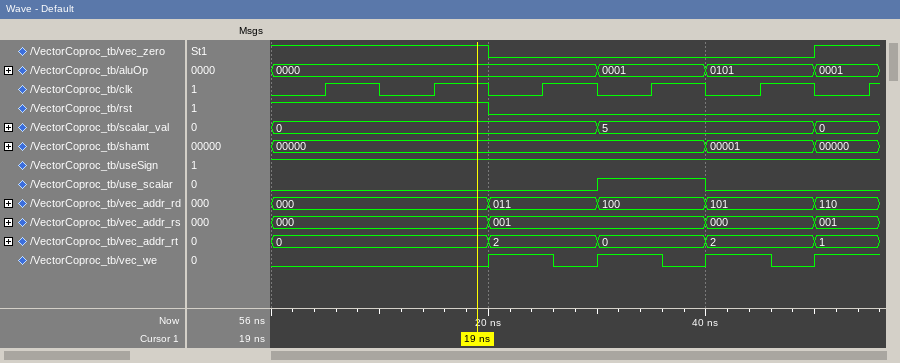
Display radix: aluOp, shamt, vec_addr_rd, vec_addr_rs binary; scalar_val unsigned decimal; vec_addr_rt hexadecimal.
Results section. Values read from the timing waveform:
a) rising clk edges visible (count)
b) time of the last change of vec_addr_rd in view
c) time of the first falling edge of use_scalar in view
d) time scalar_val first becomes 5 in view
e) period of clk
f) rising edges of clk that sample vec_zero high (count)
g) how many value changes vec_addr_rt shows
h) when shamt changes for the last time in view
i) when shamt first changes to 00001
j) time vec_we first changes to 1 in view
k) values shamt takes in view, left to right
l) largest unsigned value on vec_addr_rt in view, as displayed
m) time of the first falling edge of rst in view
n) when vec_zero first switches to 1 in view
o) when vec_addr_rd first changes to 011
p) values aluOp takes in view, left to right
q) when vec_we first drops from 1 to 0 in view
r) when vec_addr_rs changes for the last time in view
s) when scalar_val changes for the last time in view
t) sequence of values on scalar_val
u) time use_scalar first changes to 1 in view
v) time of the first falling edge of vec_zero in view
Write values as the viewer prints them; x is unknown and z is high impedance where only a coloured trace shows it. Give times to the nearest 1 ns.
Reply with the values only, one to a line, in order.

6
50 ns
40 ns
30 ns
10 ns
3
4
50 ns
40 ns
20 ns
00000, 00001, 00000
2
20 ns
50 ns
20 ns
0000, 0001, 0101, 0001
26 ns
50 ns
50 ns
0, 5, 0
30 ns
20 ns
